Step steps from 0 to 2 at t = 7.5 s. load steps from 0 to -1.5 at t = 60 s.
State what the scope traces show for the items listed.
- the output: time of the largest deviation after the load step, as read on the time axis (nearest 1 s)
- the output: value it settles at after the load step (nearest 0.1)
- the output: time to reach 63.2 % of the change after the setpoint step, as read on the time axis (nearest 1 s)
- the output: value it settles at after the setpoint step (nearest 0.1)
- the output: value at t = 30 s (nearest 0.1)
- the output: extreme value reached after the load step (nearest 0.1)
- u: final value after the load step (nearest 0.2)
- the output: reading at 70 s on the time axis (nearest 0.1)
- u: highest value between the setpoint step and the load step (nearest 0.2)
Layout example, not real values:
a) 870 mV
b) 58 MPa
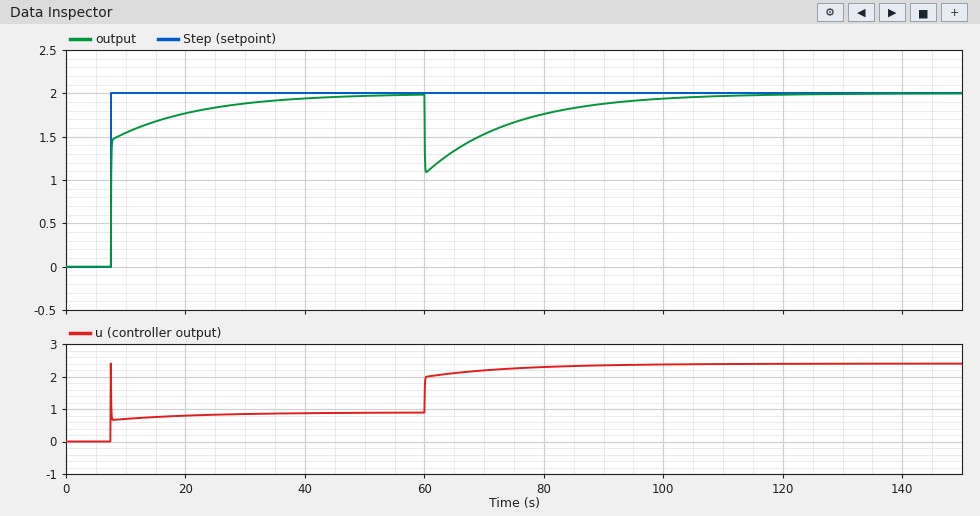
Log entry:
a) 60 s
b) 2.0
c) 8 s
d) 2.0
e) 1.9
f) 1.1
g) 2.4
h) 1.5
i) 2.4
